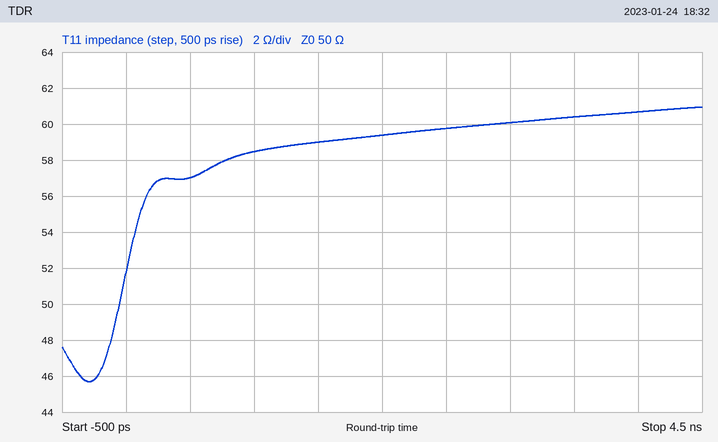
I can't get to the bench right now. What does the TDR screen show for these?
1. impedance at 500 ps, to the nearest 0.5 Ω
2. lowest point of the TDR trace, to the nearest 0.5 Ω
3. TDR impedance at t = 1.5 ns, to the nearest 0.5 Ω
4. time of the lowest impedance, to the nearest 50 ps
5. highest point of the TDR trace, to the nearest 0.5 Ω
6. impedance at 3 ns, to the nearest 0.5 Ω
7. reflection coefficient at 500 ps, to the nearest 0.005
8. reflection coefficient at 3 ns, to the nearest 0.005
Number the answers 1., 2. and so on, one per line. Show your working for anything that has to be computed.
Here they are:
1. 57.0 Ω
2. 45.5 Ω
3. 59.0 Ω
4. -300 ps
5. 61.0 Ω
6. 60.0 Ω
7. (57 − 50)/(57 + 50) ≈ +0.065
8. (60 − 50)/(60 + 50) ≈ +0.0909, so +0.090 to the nearest 0.005
